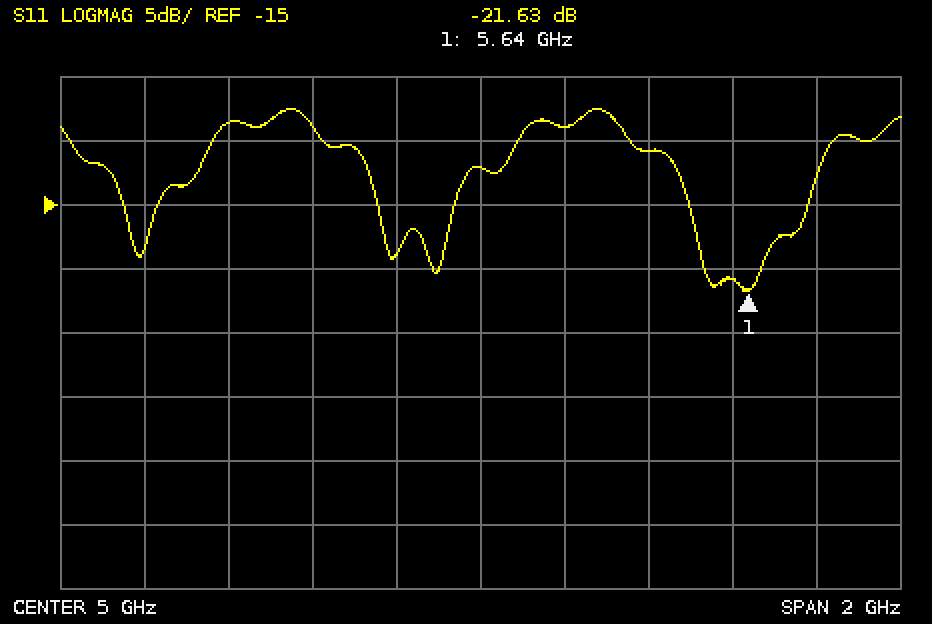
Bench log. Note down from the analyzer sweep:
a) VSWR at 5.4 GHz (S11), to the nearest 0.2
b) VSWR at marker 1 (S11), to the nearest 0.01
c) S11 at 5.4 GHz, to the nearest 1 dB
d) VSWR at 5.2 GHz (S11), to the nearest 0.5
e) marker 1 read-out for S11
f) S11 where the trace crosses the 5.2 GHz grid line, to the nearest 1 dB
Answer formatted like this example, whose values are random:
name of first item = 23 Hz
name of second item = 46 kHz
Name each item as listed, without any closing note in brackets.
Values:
VSWR at 5.4 GHz (S11), to the nearest 0.2 = 1.8
VSWR at marker 1 (S11), to the nearest 0.01 = 1.18
S11 at 5.4 GHz, to the nearest 1 dB = -11 dB
VSWR at 5.2 GHz (S11), to the nearest 0.5 = 2.0
marker 1 read-out for S11 = -21.63 dB
S11 where the trace crosses the 5.2 GHz grid line, to the nearest 1 dB = -9 dB
